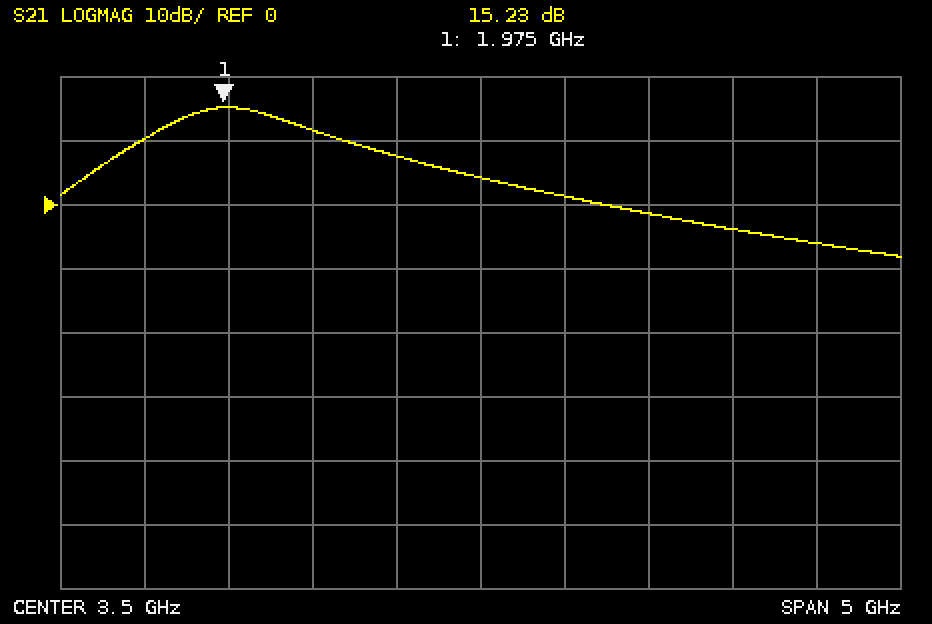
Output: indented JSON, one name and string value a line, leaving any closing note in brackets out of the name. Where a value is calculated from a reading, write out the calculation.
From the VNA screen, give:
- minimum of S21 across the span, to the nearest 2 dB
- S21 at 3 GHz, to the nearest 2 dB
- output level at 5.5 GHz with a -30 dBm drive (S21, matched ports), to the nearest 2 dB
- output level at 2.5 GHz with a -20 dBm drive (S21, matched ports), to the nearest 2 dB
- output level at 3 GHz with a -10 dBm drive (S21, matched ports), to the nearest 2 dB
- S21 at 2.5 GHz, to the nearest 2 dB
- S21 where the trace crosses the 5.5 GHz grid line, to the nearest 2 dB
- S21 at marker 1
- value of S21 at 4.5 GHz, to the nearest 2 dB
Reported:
{
  "minimum of S21 across the span, to the nearest 2 dB": "-8 dB",
  "S21 at 3 GHz, to the nearest 2 dB": "8 dB",
  "output level at 5.5 GHz with a -30 dBm drive (S21, matched ports), to the nearest 2 dB": "-30 dBm + (-6 dB) = -36 dBm",
  "output level at 2.5 GHz with a -20 dBm drive (S21, matched ports), to the nearest 2 dB": "-20 dBm + (12 dB) = -8 dBm",
  "output level at 3 GHz with a -10 dBm drive (S21, matched ports), to the nearest 2 dB": "-10 dBm + (8 dB) = -2 dBm",
  "S21 at 2.5 GHz, to the nearest 2 dB": "12 dB",
  "S21 where the trace crosses the 5.5 GHz grid line, to the nearest 2 dB": "-6 dB",
  "S21 at marker 1": "15.23 dB",
  "value of S21 at 4.5 GHz, to the nearest 2 dB": "-2 dB"
}
